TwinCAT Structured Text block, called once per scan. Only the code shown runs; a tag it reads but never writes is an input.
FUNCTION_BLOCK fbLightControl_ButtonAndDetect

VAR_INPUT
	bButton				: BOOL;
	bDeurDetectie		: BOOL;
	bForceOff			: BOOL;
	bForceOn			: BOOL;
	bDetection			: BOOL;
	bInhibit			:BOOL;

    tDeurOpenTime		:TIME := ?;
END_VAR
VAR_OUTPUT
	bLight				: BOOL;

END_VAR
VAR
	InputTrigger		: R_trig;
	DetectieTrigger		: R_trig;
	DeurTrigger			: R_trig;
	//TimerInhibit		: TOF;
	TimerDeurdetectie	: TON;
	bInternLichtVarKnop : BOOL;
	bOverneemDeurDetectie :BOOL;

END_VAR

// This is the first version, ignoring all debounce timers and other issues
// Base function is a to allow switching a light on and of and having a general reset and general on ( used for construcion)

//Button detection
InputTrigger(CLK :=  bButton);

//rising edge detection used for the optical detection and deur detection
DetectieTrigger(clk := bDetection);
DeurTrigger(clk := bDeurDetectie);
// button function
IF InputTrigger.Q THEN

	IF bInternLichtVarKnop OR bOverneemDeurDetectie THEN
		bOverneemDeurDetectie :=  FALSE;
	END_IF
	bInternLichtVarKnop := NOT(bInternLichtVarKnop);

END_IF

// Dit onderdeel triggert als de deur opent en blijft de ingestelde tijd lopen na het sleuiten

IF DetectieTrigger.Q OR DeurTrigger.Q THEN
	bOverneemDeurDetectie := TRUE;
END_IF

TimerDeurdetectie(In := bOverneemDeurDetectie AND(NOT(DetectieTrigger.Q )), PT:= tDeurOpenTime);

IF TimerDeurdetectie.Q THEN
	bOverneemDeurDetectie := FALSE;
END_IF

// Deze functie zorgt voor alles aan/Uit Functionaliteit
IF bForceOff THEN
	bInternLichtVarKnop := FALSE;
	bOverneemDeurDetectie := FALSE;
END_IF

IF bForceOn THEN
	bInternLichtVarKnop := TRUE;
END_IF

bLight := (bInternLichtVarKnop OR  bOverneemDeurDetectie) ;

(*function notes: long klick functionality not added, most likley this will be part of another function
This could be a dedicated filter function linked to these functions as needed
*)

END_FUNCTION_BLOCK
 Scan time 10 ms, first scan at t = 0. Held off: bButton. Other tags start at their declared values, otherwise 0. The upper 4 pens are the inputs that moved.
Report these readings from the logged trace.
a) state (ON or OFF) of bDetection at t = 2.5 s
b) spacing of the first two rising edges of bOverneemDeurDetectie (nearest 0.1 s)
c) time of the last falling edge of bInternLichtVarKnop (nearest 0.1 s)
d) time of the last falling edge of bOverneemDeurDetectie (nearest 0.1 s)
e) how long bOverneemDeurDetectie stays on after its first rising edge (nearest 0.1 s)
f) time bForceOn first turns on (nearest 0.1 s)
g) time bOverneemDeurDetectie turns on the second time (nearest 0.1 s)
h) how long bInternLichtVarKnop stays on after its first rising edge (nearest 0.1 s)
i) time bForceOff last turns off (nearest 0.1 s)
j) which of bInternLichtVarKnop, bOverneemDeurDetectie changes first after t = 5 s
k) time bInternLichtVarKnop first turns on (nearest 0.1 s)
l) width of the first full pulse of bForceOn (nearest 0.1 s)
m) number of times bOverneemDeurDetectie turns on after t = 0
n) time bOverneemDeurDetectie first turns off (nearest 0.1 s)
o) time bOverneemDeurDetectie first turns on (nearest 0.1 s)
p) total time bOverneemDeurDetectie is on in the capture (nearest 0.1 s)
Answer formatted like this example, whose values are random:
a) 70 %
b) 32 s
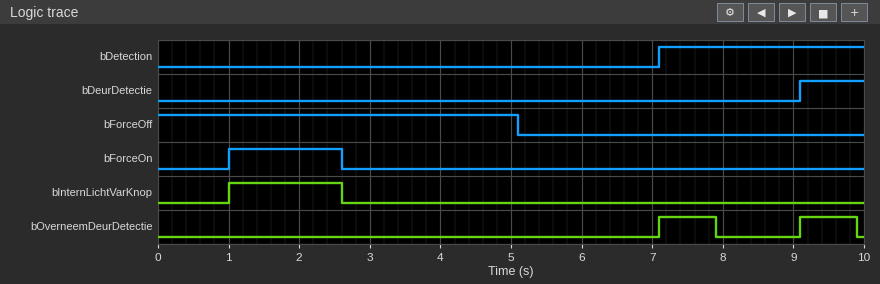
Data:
a) OFF
b) 2.0 s
c) 2.6 s
d) 9.9 s
e) 0.8 s
f) 1.0 s
g) 9.1 s
h) 1.6 s
i) 5.1 s
j) bOverneemDeurDetectie
k) 1.0 s
l) 1.6 s
m) 2
n) 7.9 s
o) 7.1 s
p) 1.6 s
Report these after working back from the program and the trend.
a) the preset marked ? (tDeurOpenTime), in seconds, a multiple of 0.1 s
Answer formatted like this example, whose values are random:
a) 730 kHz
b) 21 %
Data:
a) 0.8 s
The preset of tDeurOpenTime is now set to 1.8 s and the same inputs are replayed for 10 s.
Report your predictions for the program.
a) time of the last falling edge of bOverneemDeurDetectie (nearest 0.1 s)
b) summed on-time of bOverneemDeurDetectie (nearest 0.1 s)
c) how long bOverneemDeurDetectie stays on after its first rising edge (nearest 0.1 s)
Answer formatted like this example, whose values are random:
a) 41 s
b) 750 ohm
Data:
a) 8.9 s
b) 2.7 s
c) 1.8 s
